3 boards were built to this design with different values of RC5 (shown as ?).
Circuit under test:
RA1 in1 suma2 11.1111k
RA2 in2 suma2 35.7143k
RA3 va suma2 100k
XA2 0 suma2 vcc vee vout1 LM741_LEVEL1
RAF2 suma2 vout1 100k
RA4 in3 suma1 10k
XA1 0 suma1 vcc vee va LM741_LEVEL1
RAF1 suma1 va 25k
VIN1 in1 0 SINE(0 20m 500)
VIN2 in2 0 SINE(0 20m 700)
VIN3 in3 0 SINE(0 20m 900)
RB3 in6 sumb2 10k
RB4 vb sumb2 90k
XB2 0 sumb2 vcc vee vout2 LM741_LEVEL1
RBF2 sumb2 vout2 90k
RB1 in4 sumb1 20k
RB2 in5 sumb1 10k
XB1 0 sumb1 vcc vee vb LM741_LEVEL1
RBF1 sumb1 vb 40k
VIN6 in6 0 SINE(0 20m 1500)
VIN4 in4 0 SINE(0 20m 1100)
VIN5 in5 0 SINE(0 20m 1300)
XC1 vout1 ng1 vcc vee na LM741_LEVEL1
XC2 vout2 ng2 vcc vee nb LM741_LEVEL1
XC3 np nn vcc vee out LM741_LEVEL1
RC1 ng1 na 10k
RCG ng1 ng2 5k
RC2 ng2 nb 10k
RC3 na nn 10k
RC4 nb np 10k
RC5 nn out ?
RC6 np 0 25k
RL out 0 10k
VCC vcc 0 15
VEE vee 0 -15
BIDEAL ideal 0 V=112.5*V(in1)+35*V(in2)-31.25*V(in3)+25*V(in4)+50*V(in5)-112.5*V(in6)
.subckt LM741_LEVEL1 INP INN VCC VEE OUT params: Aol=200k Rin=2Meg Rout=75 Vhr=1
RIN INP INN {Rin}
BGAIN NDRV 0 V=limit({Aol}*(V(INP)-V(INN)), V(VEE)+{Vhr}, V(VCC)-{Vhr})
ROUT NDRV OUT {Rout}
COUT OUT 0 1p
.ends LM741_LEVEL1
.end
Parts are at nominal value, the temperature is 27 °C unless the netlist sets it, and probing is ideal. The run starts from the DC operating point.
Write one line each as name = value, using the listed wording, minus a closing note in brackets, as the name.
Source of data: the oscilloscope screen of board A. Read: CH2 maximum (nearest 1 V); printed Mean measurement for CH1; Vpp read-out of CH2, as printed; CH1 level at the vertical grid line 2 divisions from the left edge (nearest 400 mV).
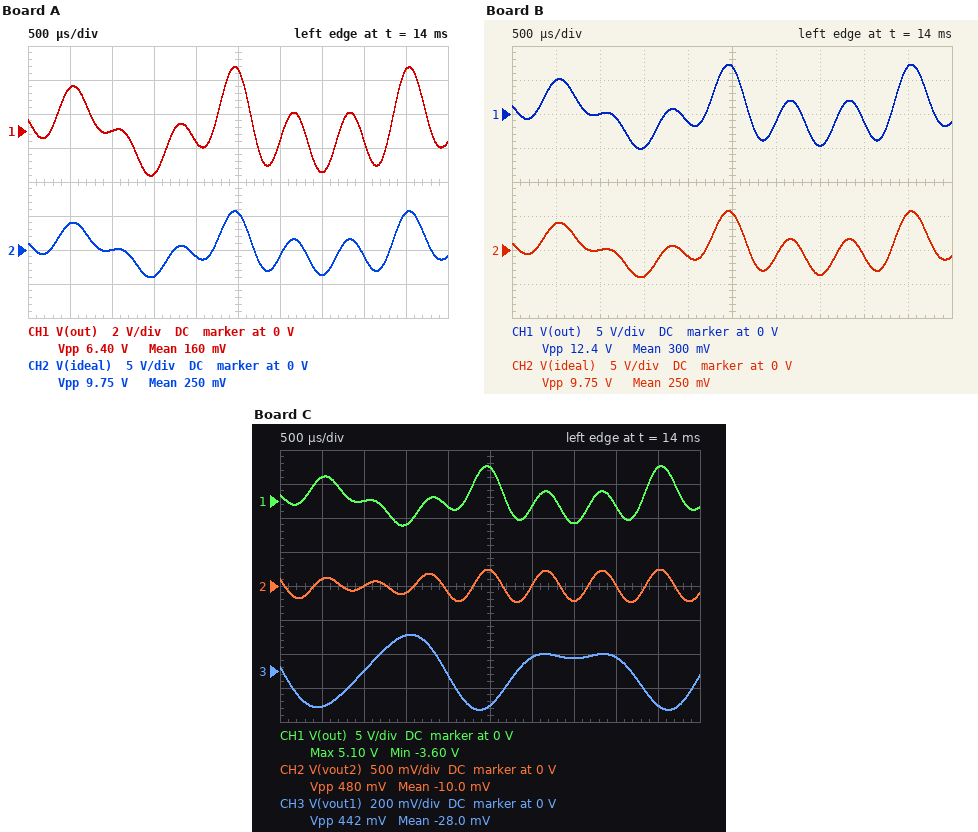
CH2 maximum = 6 V
printed Mean measurement for CH1 = 160 mV
Vpp read-out of CH2, as printed = 9.75 V
CH1 level at the vertical grid line 2 divisions from the left edge = 0 V
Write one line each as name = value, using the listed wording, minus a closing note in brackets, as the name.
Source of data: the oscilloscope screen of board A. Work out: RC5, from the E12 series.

RC5, from the E12 series = 15 kΩ
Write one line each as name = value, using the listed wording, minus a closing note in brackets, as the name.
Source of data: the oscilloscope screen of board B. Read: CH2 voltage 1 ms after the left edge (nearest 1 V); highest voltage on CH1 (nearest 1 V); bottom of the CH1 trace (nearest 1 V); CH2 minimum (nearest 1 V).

CH2 voltage 1 ms after the left edge = 0 V
highest voltage on CH1 = 7 V
bottom of the CH1 trace = -5 V
CH2 minimum = -4 V
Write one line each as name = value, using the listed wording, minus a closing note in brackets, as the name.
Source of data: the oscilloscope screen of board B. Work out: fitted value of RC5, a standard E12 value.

fitted value of RC5, a standard E12 value = 33 kΩ
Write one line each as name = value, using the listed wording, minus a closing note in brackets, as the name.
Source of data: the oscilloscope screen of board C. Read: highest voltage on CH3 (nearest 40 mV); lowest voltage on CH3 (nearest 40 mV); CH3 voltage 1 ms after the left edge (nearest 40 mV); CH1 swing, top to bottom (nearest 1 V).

highest voltage on CH3 = 200 mV
lowest voltage on CH3 = -240 mV
CH3 voltage 1 ms after the left edge = 0 V
CH1 swing, top to bottom = 9 V
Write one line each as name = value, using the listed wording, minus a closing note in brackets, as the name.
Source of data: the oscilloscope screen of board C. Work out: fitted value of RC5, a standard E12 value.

fitted value of RC5, a standard E12 value = 22 kΩ
